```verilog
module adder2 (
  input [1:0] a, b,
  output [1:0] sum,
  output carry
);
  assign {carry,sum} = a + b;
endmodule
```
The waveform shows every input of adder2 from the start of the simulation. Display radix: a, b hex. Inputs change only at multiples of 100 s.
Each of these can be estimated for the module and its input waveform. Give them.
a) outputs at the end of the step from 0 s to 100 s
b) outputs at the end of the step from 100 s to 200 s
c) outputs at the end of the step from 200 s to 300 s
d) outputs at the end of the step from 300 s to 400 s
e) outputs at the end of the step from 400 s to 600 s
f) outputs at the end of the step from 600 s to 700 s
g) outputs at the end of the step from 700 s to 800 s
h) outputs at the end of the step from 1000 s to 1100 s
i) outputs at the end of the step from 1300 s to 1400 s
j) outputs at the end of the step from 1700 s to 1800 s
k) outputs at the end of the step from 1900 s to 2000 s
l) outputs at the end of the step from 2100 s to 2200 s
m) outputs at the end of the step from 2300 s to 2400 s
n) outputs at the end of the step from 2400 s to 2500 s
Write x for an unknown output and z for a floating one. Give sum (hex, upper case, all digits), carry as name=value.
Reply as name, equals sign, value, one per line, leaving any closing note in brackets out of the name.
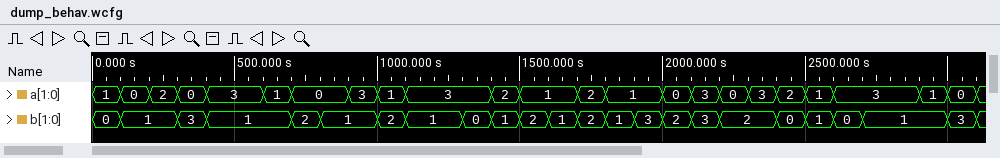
outputs at the end of the step from 0 s to 100 s = sum=1, carry=0
outputs at the end of the step from 100 s to 200 s = sum=1, carry=0
outputs at the end of the step from 200 s to 300 s = sum=3, carry=0
outputs at the end of the step from 300 s to 400 s = sum=3, carry=0
outputs at the end of the step from 400 s to 600 s = sum=0, carry=1
outputs at the end of the step from 600 s to 700 s = sum=2, carry=0
outputs at the end of the step from 700 s to 800 s = sum=2, carry=0
outputs at the end of the step from 1000 s to 1100 s = sum=3, carry=0
outputs at the end of the step from 1300 s to 1400 s = sum=3, carry=0
outputs at the end of the step from 1700 s to 1800 s = sum=0, carry=1
outputs at the end of the step from 1900 s to 2000 s = sum=0, carry=1
outputs at the end of the step from 2100 s to 2200 s = sum=2, carry=1
outputs at the end of the step from 2300 s to 2400 s = sum=1, carry=1
outputs at the end of the step from 2400 s to 2500 s = sum=2, carry=0
